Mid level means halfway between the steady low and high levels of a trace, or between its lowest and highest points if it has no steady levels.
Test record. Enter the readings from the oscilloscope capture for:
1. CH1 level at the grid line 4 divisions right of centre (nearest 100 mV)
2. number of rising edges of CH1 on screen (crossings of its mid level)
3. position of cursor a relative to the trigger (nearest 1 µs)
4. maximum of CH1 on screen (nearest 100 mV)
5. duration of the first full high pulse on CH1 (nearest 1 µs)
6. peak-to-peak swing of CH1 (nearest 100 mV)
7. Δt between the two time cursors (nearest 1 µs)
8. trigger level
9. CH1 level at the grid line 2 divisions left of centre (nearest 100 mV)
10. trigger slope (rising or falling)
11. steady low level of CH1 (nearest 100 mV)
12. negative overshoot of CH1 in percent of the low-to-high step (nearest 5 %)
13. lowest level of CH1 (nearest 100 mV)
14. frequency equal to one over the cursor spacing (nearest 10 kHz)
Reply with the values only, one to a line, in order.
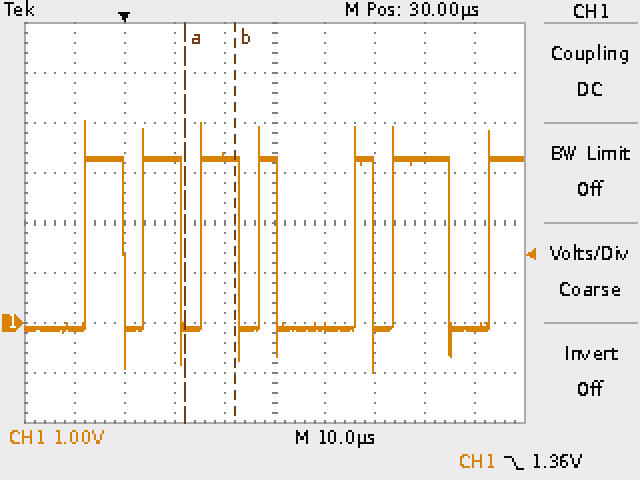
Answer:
-100 mV
7
+12 µs
4.0 V
8 µs
5.0 V
10 µs
1.36 V
3.3 V
falling
-100 mV
25 %
-1.0 V
100 kHz
